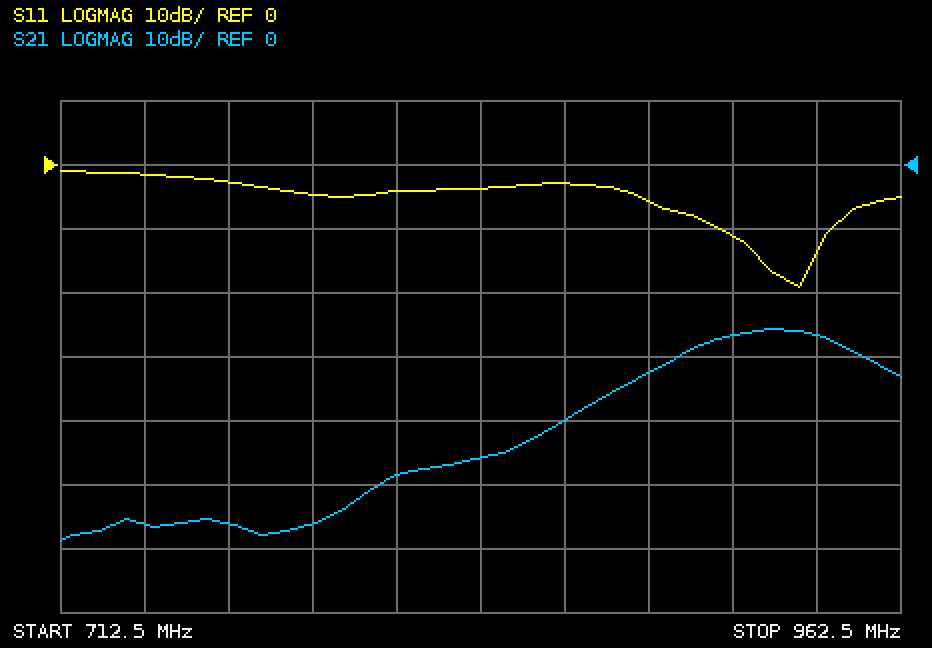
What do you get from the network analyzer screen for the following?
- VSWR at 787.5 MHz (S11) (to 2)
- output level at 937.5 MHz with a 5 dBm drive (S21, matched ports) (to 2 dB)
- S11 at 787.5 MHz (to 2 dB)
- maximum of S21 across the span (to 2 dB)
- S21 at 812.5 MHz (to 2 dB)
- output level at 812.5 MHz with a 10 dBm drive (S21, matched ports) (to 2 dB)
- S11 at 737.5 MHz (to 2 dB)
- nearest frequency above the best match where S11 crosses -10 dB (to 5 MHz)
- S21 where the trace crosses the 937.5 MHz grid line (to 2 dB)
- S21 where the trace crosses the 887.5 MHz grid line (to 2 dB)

4
-22 dBm
-4 dB
-26 dB
-48 dB
-38 dBm
-2 dB
940 MHz
-26 dB
-32 dB
